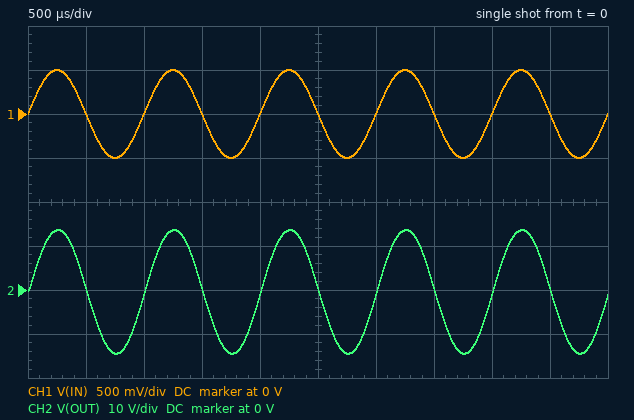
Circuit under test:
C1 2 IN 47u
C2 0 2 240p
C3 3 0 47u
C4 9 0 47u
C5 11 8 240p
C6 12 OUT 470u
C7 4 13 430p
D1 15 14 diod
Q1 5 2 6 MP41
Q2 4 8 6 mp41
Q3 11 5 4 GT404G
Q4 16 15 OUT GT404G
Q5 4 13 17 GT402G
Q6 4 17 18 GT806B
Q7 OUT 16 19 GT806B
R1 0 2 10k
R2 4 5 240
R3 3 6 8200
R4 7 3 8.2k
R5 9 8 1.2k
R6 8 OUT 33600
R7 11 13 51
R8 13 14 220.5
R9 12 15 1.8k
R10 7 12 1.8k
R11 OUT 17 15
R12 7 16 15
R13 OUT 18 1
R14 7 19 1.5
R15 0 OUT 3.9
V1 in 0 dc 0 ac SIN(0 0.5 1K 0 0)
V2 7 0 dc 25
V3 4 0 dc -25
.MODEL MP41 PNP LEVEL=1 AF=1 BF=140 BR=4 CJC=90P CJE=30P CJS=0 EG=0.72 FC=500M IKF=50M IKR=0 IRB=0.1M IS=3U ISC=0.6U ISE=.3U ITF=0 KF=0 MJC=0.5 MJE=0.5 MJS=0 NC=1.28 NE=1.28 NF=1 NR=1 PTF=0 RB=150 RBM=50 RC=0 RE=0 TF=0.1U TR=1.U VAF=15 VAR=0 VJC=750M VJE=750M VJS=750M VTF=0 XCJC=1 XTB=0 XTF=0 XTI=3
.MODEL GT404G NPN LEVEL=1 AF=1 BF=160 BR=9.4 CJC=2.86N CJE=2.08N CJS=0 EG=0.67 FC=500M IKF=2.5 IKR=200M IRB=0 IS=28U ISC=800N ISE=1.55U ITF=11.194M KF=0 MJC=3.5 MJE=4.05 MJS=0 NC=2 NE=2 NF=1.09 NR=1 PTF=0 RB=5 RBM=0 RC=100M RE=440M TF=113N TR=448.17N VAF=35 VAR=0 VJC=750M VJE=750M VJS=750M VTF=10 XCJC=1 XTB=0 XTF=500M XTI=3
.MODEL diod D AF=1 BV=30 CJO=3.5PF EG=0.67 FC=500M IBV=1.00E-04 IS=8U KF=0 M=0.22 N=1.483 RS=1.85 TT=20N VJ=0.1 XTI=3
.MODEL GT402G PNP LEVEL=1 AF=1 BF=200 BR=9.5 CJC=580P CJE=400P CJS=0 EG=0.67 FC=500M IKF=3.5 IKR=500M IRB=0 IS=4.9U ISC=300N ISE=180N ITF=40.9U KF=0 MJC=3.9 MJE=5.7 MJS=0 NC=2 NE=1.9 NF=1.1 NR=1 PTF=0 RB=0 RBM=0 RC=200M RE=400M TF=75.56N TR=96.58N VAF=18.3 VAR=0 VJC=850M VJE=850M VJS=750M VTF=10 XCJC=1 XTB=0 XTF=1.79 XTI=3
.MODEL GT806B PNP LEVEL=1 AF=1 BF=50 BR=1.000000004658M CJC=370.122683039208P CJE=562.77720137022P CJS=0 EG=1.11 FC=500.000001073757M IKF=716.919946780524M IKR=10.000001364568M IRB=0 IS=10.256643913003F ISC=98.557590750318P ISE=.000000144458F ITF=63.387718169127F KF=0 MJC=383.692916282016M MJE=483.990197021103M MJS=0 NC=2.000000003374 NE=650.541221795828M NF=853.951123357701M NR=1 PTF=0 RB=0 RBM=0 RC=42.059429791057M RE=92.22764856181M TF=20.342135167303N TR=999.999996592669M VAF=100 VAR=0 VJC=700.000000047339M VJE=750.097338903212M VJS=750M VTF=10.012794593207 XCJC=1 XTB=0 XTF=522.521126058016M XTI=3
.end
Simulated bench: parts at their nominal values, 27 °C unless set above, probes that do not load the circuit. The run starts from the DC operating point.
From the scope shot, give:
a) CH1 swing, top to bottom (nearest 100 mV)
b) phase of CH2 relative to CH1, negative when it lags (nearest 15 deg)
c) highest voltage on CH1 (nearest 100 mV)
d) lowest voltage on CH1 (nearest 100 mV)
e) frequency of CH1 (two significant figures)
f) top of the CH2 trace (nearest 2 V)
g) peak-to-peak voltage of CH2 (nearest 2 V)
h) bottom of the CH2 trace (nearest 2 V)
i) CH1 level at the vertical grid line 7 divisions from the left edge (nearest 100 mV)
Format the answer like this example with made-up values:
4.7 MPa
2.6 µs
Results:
1.0 V
0 deg
500 mV
-500 mV
1.0 kHz
14 V
28 V
-14 V
0 V
